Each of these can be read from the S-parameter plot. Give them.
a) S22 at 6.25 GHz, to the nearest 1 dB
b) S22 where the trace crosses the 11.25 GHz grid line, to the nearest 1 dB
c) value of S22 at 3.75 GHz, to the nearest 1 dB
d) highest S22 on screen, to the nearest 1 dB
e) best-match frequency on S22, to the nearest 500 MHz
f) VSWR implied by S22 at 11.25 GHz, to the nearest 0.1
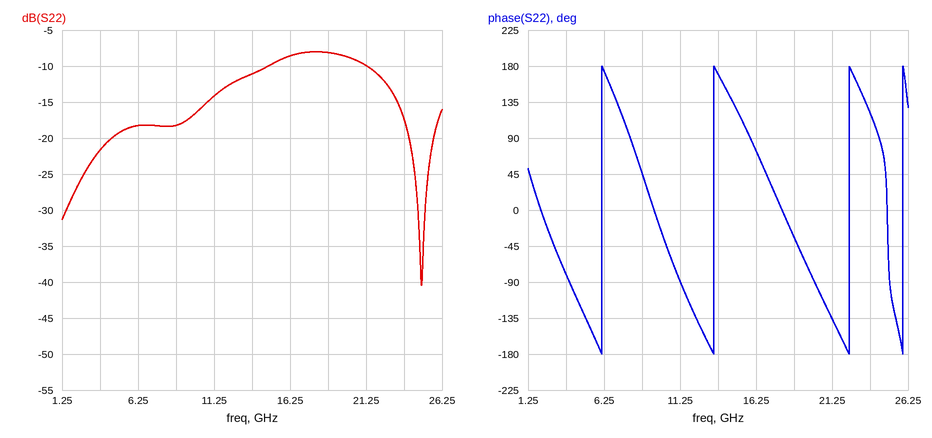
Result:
-18 dB
-14 dB
-22 dB
-8 dB
25.0 GHz
1.5
